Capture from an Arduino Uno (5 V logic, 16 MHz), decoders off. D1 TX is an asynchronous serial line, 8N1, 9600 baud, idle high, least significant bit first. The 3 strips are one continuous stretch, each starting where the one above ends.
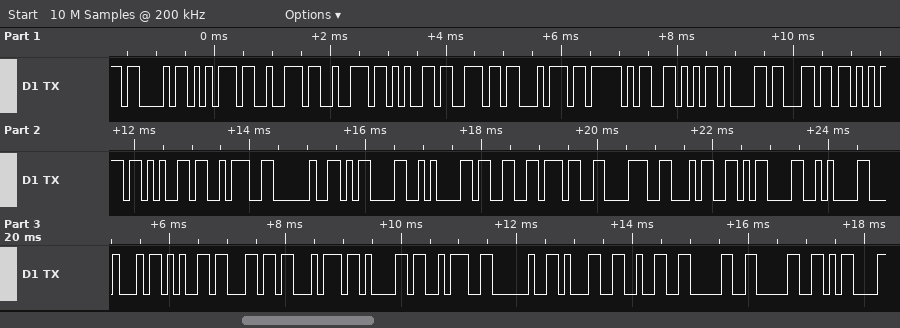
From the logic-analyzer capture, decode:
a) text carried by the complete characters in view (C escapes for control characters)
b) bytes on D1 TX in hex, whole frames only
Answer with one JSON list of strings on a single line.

["\"Current_Value: \\r\\n3784\\r\\nDelta: 1200\\r\"", "43 75 72 72 65 6E 74 5F 56 61 6C 75 65 3A 20 0D 0A 33 37 38 34 0D 0A 44 65 6C 74 61 3A 20 31 32 30 30 0D"]
